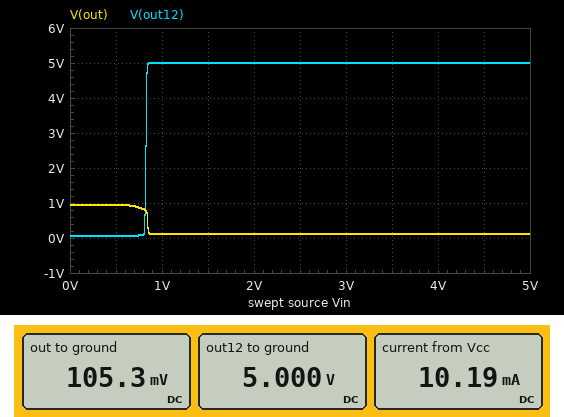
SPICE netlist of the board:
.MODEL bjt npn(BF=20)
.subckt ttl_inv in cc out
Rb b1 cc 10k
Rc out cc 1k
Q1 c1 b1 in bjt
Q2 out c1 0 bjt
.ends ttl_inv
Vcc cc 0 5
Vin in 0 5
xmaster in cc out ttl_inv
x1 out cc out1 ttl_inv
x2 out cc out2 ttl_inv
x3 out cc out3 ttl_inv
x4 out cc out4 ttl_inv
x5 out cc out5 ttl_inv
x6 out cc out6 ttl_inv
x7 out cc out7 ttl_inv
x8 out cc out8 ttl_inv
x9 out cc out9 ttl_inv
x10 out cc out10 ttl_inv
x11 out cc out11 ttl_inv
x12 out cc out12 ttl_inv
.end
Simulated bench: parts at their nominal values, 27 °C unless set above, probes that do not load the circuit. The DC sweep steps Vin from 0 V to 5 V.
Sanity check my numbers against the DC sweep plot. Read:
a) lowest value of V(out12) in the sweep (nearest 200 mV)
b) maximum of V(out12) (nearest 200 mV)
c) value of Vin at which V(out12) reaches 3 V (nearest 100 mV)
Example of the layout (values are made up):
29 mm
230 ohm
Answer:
0 V
5.0 V
800 mV
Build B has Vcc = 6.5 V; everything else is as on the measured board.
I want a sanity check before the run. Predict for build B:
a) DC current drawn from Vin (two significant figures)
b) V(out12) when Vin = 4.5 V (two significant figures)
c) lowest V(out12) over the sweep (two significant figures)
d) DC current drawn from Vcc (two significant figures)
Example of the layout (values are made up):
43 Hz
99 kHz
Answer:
490 µA
6.5 V
67 mV
14 mA
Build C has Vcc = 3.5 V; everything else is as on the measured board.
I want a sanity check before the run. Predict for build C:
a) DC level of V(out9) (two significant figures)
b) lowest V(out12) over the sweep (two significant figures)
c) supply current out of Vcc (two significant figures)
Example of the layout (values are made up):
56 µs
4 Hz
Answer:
3.5 V
76 mV
6.7 mA
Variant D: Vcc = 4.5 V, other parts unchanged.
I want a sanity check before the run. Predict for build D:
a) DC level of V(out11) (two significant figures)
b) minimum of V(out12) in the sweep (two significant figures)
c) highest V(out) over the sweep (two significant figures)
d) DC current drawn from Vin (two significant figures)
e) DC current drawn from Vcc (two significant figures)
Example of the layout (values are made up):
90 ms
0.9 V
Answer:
4.5 V
71 mV
980 mV
290 µA
9.0 mA
